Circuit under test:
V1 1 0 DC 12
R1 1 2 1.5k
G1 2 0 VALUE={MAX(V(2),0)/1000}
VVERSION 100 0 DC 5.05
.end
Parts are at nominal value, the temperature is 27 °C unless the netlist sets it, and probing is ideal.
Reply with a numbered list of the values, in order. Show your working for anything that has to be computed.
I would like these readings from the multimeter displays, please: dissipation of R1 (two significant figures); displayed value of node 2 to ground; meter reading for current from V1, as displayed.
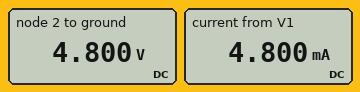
1. (12 V - 4.8 V)^2 / 1.5 kΩ = 35 mW
2. 4.800 V
3. 4.800 mA
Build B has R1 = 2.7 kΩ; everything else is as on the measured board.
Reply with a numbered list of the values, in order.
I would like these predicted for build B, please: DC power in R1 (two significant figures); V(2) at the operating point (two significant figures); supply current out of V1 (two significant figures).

1. 28 mW
2. 3.2 V
3. 3.2 mA
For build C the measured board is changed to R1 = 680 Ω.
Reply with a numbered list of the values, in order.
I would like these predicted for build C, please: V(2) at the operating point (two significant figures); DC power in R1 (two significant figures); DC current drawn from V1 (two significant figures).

1. 7.1 V
2. 35 mW
3. 7.1 mA
